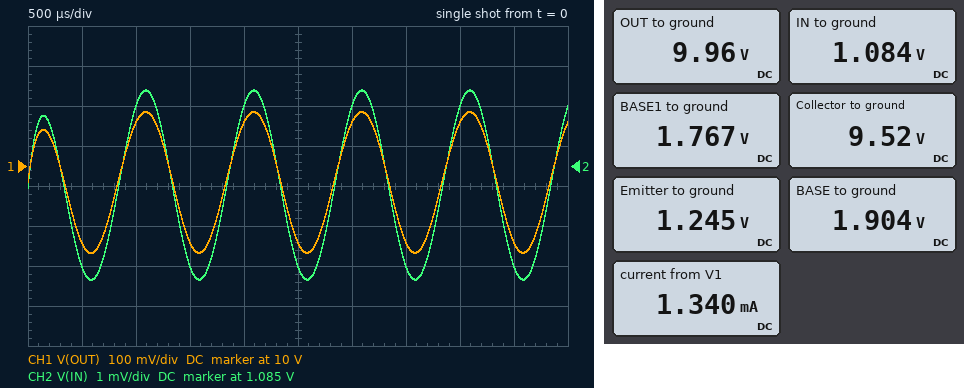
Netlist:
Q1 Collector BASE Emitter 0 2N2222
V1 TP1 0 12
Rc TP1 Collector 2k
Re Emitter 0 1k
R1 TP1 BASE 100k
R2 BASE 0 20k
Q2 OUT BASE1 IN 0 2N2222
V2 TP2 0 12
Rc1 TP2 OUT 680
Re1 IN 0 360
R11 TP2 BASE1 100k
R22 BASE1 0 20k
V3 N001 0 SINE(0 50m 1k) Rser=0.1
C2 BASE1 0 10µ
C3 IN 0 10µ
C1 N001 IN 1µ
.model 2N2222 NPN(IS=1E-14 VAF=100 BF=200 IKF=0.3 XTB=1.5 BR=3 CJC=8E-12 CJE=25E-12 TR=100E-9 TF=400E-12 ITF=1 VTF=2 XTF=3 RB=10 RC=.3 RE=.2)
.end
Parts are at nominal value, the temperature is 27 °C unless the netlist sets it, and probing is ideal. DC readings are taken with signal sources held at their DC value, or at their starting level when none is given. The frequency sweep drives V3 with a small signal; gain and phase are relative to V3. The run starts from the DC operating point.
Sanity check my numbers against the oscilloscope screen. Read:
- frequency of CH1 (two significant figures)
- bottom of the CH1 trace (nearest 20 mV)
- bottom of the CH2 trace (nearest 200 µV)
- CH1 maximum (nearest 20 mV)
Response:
1.0 kHz
9.78 V
1.0822 V
10.14 V
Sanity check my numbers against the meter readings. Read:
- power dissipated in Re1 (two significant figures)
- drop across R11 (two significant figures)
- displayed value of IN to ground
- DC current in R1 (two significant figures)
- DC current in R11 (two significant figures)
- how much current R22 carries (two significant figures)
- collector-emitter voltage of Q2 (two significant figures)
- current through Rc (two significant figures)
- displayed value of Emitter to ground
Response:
3.3 mW
10 V
1.084 V
100 µA
100 µA
88 µA
8.9 V
1.2 mA
1.245 V
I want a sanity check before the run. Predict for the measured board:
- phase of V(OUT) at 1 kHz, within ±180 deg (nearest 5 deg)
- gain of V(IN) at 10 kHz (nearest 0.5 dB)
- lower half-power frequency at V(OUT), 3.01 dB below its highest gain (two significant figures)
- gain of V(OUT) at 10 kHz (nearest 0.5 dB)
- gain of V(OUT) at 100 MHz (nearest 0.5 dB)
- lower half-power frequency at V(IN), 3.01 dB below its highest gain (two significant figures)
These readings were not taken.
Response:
60 deg
-21.0 dB
1.6 kHz
16.5 dB
-30.0 dB
1.6 kHz
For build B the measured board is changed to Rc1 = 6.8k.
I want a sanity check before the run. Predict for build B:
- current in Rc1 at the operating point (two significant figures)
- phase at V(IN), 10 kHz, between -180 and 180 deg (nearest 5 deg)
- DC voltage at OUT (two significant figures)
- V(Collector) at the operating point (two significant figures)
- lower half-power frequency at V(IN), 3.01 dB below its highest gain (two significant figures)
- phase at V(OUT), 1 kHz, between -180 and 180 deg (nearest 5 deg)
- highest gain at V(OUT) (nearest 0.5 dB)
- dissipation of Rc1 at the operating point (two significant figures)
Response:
1.7 mA
0 deg
690 mV
9.5 V
360 Hz
25 deg
0 dB
19 mW
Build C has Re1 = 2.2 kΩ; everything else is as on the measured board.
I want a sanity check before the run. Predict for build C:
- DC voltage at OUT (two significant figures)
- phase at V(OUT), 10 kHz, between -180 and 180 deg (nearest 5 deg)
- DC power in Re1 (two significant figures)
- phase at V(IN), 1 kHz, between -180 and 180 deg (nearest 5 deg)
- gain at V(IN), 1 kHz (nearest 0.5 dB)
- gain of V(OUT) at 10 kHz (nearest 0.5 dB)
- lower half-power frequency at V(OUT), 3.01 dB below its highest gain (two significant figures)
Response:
12 V
0 deg
790 µW
20 deg
-21.5 dB
3.0 dB
340 Hz
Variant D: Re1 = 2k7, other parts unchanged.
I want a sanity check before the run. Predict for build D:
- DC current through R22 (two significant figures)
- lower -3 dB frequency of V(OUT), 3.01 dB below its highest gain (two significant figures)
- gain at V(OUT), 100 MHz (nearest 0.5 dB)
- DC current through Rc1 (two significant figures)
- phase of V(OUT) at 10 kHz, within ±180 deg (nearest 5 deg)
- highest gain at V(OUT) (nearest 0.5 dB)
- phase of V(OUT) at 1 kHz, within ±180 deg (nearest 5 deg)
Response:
98 µA
280 Hz
-40.5 dB
490 µA
0 deg
1.5 dB
15 deg
